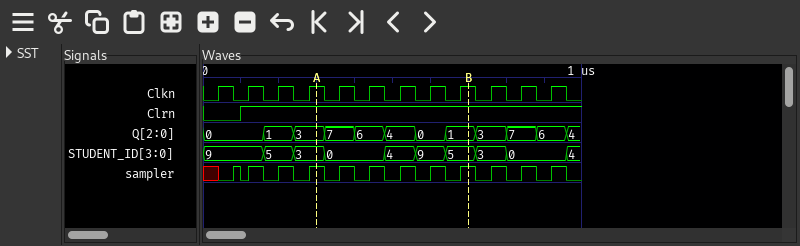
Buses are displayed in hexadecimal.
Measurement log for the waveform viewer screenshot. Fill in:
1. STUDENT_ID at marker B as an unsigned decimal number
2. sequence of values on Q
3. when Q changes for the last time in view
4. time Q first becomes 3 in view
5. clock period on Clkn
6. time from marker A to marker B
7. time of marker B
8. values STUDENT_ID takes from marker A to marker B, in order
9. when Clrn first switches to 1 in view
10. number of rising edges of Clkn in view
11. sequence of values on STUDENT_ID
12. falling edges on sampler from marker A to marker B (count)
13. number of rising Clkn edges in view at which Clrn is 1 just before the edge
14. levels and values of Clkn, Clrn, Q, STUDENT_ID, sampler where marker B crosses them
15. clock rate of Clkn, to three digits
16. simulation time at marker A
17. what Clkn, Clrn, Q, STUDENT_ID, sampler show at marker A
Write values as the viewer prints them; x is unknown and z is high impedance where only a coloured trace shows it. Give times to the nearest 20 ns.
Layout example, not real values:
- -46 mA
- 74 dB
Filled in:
- 5
- 0, 1, 3, 7, 6, 4, 0, 1, 3, 7, 6, 4
- 960 ns
- 240 ns
- 80 ns
- 400 ns
- 700 ns
- 3, 0, 4, 9, 5
- 100 ns
- 12
- 9, 5, 3, 0, 4, 9, 5, 3, 0, 4
- 5
- 11
- Clkn=1, Clrn=1, Q=1, STUDENT_ID=5, sampler=1
- 12.5 MHz
- 300 ns
- Clkn=1, Clrn=1, Q=3, STUDENT_ID=3, sampler=1
